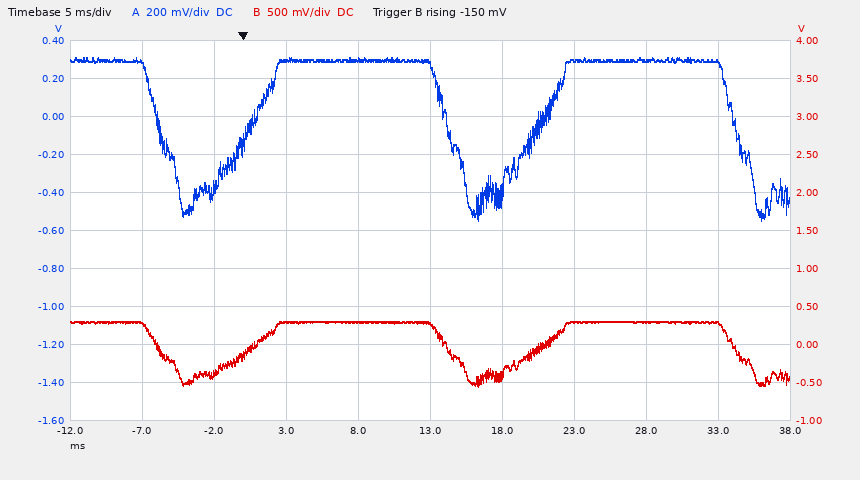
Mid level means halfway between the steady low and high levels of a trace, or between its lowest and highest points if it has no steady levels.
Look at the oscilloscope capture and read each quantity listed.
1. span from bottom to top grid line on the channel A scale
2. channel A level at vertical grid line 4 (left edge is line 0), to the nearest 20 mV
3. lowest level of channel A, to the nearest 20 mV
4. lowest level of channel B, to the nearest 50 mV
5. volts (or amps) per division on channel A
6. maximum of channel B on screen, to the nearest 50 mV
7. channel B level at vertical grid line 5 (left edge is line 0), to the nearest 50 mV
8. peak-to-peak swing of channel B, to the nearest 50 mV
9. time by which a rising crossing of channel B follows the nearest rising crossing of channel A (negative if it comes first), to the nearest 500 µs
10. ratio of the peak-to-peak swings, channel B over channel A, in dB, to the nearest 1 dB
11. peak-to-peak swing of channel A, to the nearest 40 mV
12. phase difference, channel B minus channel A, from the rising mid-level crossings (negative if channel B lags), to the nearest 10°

2 V
300 mV
-540 mV
-550 mV
200 mV
300 mV
250 mV
850 mV
0.0 ms
0 dB
840 mV
0°
